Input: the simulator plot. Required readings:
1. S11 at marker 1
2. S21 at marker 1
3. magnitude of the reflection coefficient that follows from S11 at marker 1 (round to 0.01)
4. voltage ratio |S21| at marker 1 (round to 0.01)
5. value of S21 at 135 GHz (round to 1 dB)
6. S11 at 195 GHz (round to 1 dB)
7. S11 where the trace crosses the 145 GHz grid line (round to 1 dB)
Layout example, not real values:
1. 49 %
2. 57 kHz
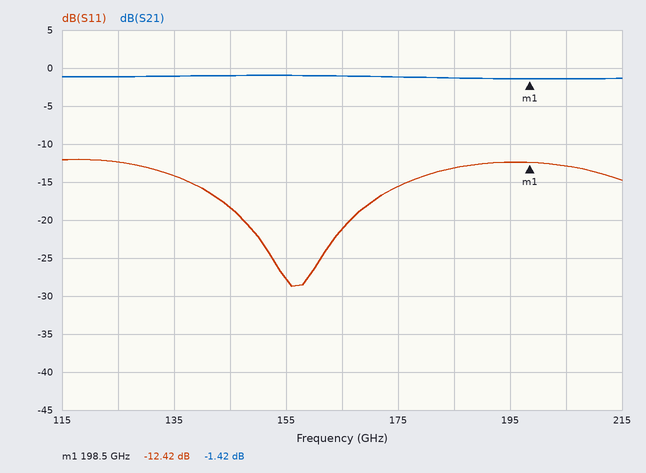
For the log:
1. -12.42 dB
2. -1.42 dB
3. 0.24
4. 0.85
5. -1 dB
6. -12 dB
7. -18 dB
